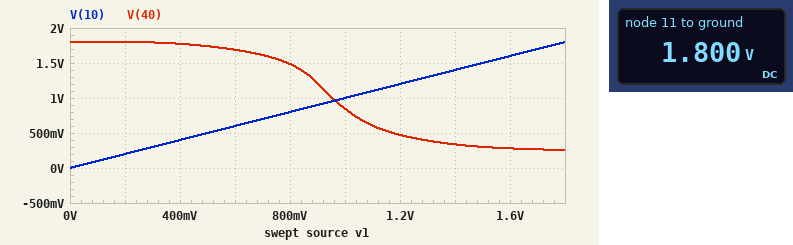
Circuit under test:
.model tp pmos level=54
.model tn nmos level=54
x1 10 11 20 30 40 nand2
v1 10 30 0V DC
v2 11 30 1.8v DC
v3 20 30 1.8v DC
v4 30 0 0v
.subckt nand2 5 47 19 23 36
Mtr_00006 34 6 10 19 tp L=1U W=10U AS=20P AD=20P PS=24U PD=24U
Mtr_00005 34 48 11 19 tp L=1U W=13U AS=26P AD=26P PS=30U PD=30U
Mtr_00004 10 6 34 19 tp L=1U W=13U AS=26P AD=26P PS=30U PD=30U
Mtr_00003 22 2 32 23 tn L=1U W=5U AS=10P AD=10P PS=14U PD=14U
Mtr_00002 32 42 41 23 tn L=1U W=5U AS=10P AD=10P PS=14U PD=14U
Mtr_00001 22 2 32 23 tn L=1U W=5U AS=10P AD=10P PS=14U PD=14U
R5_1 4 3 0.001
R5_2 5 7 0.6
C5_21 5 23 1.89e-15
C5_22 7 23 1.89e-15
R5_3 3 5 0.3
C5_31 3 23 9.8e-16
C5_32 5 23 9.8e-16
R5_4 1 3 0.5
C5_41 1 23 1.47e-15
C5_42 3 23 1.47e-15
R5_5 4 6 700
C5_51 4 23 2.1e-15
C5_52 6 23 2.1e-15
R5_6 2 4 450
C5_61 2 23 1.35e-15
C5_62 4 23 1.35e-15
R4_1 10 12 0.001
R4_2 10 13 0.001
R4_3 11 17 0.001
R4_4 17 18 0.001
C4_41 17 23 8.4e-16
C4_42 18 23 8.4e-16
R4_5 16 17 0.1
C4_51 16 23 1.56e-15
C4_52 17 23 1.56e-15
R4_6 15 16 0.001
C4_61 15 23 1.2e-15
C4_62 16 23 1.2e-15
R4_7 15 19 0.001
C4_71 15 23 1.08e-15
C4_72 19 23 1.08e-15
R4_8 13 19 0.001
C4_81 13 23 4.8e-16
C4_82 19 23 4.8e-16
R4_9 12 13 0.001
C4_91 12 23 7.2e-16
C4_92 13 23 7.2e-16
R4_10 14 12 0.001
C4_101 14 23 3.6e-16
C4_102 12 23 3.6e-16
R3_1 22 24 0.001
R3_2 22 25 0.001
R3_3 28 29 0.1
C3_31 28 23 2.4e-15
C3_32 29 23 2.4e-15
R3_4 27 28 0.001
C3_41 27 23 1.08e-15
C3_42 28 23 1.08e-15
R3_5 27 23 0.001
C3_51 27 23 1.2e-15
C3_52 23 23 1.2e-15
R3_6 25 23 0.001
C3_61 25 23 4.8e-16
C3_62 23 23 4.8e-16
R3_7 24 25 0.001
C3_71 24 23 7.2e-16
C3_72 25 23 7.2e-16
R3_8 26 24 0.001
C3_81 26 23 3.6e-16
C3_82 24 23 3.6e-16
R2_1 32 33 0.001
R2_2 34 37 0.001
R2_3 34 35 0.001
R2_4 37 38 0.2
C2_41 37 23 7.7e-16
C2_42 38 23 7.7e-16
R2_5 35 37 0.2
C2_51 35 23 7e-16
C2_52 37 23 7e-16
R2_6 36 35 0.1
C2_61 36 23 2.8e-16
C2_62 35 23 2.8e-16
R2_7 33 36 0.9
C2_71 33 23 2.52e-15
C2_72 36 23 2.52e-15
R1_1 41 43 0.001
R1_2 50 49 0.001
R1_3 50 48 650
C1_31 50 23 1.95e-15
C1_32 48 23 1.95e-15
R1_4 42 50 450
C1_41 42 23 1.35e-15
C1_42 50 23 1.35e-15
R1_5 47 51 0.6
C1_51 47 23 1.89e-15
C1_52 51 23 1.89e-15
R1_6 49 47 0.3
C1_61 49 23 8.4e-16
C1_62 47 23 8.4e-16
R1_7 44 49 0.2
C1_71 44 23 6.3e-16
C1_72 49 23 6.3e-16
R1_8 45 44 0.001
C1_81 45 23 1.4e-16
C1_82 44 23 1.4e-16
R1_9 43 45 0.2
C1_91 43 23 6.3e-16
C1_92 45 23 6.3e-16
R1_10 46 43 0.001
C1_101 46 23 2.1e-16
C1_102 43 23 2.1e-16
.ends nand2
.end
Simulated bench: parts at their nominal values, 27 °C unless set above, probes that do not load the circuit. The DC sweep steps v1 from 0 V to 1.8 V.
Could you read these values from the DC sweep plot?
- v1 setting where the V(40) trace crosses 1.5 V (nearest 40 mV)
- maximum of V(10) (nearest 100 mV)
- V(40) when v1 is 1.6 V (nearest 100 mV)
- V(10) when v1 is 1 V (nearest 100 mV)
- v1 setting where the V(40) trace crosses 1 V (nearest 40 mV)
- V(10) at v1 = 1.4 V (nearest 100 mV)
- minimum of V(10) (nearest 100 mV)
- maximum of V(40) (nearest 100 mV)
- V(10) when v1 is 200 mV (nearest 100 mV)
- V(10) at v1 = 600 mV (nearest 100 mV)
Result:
800 mV
1.8 V
300 mV
1.0 V
960 mV
1.4 V
0 V
1.8 V
200 mV
600 mV
